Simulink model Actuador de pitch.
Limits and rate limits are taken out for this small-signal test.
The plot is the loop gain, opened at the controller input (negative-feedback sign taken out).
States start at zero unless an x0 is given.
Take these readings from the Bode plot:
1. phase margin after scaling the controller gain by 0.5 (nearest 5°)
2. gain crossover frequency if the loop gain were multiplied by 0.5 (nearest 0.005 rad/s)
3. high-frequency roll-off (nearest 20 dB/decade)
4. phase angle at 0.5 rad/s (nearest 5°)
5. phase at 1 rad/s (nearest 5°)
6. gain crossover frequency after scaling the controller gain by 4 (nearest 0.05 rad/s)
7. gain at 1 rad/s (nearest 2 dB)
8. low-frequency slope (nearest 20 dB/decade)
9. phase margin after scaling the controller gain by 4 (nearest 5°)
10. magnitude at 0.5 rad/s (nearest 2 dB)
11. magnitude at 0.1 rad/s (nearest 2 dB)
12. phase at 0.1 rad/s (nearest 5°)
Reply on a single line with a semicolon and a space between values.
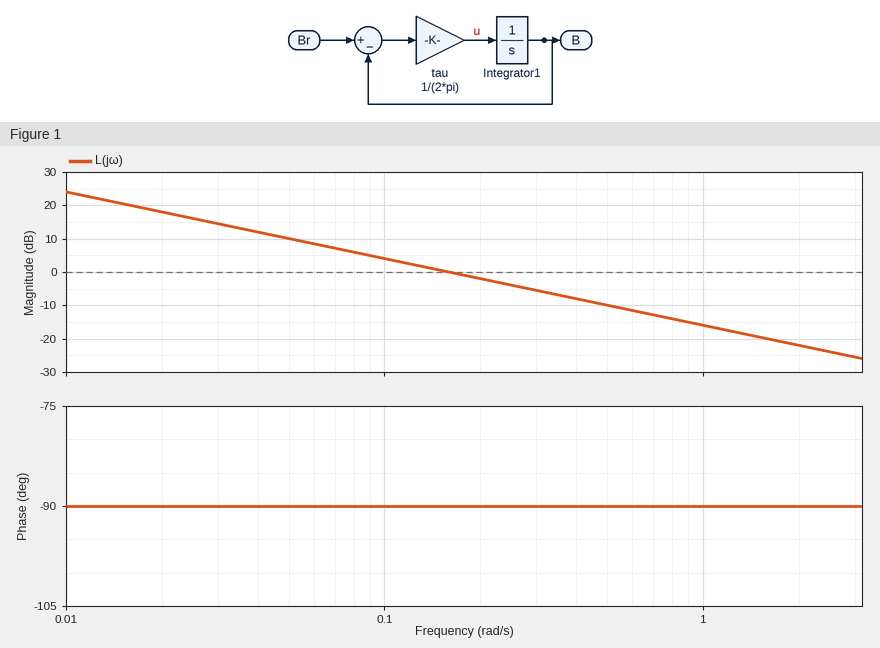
90°; 0.080 rad/s; -20 dB/decade; -90°; -90°; 0.65 rad/s; -16 dB; -20 dB/decade; 90°; -10 dB; 4 dB; -90°
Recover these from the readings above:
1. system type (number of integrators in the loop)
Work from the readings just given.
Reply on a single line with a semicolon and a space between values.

1
